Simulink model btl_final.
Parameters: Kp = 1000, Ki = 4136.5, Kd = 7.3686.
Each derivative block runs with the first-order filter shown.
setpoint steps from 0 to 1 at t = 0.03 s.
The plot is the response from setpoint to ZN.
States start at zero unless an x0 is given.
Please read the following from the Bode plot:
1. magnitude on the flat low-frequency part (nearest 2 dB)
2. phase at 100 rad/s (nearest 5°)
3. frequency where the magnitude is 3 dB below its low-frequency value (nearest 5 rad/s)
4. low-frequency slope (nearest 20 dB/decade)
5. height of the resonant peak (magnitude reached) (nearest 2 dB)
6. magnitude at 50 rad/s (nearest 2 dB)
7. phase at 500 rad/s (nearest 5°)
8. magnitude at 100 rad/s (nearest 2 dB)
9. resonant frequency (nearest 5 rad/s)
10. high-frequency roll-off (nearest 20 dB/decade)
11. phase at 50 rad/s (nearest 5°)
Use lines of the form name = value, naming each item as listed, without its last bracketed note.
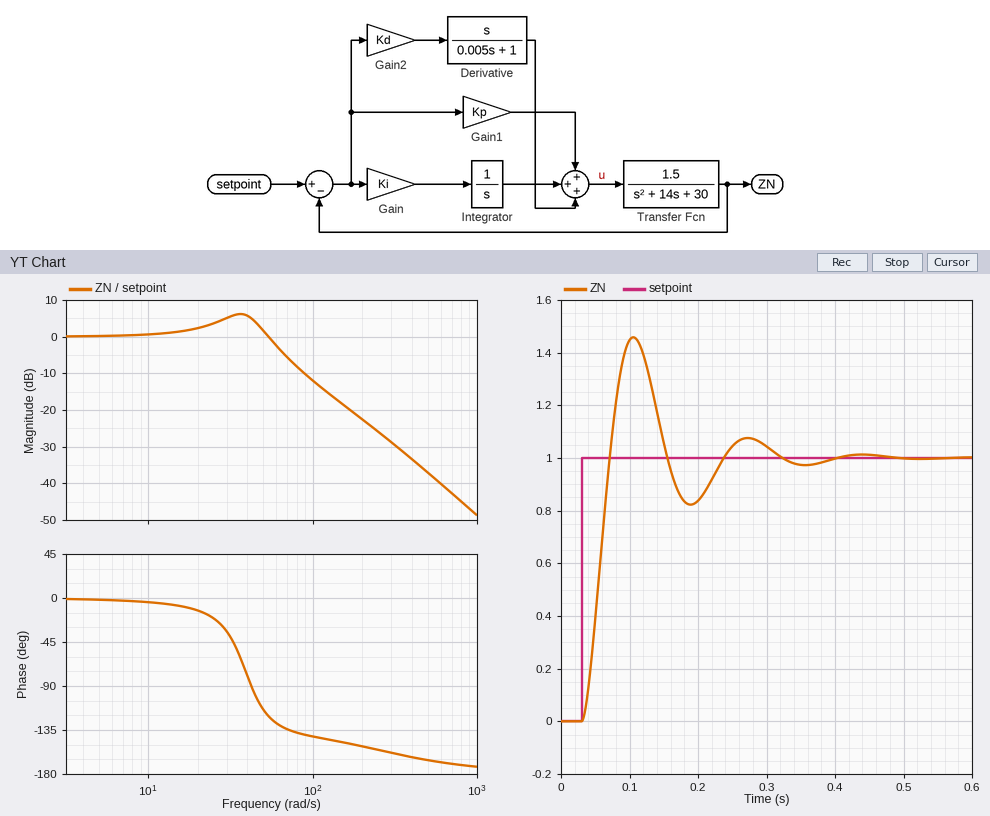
magnitude on the flat low-frequency part = 0 dB
phase at 100 rad/s = -140°
frequency where the magnitude is 3 dB below its low-frequency value = 60 rad/s
low-frequency slope = 0 dB/decade
height of the resonant peak (magnitude reached) = 6 dB
magnitude at 50 rad/s = 2 dB
phase at 500 rad/s = -165°
magnitude at 100 rad/s = -12 dB
resonant frequency = 35 rad/s
high-frequency roll-off = -40 dB/decade
phase at 50 rad/s = -115°
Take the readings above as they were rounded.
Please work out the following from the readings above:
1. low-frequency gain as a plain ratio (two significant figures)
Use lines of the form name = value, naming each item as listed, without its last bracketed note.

low-frequency gain as a plain ratio = 1.0
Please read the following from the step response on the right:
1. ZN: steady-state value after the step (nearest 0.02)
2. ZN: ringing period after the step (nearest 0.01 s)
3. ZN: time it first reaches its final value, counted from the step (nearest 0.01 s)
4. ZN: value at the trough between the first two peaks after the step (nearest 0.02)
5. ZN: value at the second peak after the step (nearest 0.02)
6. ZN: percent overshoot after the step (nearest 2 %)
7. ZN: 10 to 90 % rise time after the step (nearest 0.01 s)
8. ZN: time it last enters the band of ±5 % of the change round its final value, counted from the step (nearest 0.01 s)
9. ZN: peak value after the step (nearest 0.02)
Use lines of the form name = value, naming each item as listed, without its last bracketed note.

ZN: steady-state value after the step = 1.00
ZN: ringing period after the step = 0.17 s
ZN: time it first reaches its final value, counted from the step = 0.04 s
ZN: value at the trough between the first two peaks after the step = 0.82
ZN: value at the second peak after the step = 1.08
ZN: percent overshoot after the step = 46 %
ZN: 10 to 90 % rise time after the step = 0.03 s
ZN: time it last enters the band of ±5 % of the change round its final value, counted from the step = 0.27 s
ZN: peak value after the step = 1.46
